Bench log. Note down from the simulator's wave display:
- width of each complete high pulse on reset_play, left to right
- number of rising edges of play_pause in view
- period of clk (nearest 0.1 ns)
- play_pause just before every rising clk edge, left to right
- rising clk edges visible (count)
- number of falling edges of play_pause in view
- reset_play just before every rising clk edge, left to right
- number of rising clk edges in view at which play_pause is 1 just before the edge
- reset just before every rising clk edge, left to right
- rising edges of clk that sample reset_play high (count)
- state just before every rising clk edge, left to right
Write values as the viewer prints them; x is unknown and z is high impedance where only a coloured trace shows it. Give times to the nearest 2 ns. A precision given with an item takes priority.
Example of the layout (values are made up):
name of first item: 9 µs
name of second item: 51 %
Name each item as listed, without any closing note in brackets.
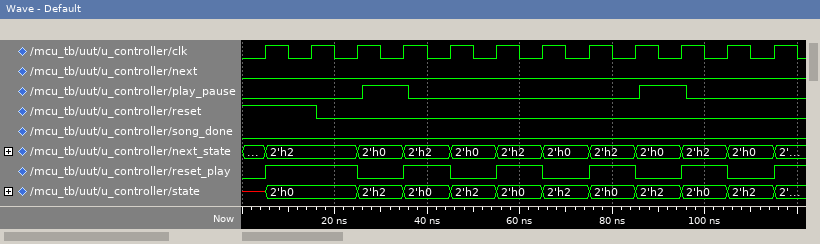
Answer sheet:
width of each complete high pulse on reset_play, left to right: 20 ns, 10 ns, 10 ns, 10 ns, 10 ns
number of rising edges of play_pause in view: 2
period of clk: 10 ns
play_pause just before every rising clk edge, left to right: 0 0 0 1 0 0 0 0 0 1 0 0
rising clk edges visible: 12
number of falling edges of play_pause in view: 2
reset_play just before every rising clk edge, left to right: 0 1 1 0 1 0 1 0 1 0 1 0
number of rising clk edges in view at which play_pause is 1 just before the edge: 2
reset just before every rising clk edge, left to right: 1 1 0 0 0 0 0 0 0 0 0 0
rising edges of clk that sample reset_play high: 6
state just before every rising clk edge, left to right: x, 2'h0, 2'h0, 2'h2, 2'h0, 2'h2, 2'h0, 2'h2, 2'h0, 2'h2, 2'h0, 2'h2
